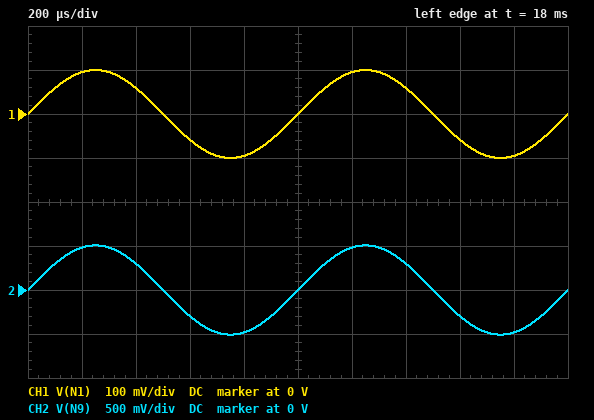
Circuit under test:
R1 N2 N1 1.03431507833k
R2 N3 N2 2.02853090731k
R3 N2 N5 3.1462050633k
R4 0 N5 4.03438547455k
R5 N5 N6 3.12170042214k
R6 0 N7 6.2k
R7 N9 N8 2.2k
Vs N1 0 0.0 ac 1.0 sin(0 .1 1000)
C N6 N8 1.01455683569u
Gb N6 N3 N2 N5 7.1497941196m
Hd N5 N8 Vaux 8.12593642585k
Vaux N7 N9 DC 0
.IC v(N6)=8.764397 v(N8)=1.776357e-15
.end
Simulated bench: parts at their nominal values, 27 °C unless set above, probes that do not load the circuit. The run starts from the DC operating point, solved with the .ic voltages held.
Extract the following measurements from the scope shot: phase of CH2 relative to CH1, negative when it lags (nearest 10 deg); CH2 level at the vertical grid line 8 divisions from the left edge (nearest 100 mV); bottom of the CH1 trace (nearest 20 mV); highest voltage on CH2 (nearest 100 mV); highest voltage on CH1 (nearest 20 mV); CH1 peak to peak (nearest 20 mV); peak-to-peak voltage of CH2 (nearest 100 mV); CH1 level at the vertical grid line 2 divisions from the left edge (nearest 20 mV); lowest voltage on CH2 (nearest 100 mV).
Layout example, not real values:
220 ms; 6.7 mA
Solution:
0 deg; -300 mV; -100 mV; 500 mV; 100 mV; 200 mV; 1.0 V; 60 mV; -500 mV
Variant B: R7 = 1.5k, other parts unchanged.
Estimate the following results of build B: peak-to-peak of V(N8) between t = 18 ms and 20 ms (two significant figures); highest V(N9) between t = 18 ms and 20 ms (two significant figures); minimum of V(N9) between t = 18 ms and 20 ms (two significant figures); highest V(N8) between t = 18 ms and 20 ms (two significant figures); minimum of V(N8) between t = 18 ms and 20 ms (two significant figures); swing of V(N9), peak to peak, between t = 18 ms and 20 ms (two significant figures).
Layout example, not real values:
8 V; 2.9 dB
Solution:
4.2 V; 1.7 V; -1.7 V; 2.1 V; -2.1 V; 3.4 V
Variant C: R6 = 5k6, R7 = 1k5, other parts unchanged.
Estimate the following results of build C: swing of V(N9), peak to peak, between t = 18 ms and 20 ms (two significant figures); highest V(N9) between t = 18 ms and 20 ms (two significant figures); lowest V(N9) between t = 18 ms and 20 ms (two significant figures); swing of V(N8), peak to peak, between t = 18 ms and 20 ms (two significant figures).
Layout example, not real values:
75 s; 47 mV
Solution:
3.1 V; 1.5 V; -1.5 V; 3.9 V
